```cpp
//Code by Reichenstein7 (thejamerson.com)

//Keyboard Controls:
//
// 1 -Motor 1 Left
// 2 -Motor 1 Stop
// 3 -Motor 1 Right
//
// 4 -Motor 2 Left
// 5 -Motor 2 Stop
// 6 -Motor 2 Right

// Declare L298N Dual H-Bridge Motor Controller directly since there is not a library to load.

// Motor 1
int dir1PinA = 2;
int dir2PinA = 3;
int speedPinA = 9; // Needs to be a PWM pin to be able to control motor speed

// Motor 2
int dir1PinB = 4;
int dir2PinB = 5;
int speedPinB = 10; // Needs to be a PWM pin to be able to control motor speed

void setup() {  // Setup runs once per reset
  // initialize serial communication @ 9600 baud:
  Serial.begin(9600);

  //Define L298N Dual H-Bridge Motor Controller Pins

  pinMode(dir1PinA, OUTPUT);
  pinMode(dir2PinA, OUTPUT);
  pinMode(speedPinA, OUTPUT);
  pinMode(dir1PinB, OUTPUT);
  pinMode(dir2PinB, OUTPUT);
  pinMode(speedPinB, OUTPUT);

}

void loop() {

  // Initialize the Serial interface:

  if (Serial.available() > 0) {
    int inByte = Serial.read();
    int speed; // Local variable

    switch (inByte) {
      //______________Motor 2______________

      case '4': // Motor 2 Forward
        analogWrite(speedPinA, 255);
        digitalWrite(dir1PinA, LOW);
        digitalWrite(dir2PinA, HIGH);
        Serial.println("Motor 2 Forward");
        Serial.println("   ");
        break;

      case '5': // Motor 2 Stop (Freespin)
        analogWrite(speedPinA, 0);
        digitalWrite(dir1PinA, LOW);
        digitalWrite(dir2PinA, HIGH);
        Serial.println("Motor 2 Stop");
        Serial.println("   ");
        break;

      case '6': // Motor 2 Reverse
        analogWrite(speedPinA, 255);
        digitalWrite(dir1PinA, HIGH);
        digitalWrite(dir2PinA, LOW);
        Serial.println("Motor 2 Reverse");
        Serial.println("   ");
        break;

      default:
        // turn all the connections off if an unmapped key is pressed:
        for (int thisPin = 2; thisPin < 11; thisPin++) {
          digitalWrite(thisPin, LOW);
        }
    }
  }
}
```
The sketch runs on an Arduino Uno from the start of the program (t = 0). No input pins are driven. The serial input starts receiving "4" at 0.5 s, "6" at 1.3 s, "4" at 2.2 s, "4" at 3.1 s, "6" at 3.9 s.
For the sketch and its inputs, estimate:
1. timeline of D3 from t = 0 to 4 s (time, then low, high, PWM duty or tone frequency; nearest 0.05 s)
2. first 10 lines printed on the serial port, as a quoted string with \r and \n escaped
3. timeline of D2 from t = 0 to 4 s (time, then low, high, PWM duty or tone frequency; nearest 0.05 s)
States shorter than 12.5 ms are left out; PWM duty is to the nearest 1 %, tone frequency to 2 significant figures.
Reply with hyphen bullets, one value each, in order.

- 0 s low; 0.5 s high; 1.3 s low; 2.2 s high; 3.9 s low
- "Motor 2 Forward\r\n   \r\nMotor 2 Reverse\r\n   \r\nMotor 2 Forward\r\n   \r\nMotor 2 Forward\r\n   \r\nMotor 2 Reverse\r\n   \r\n"
- 0 s low; 1.3 s high; 2.2 s low; 3.9 s high
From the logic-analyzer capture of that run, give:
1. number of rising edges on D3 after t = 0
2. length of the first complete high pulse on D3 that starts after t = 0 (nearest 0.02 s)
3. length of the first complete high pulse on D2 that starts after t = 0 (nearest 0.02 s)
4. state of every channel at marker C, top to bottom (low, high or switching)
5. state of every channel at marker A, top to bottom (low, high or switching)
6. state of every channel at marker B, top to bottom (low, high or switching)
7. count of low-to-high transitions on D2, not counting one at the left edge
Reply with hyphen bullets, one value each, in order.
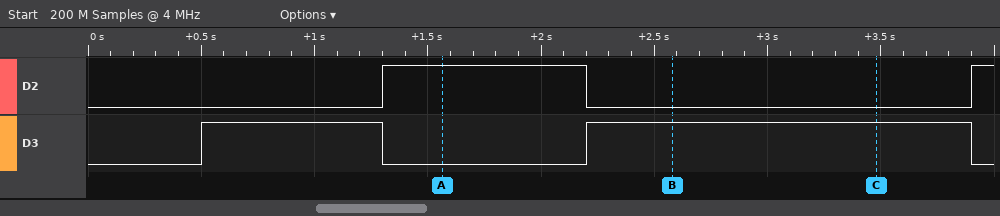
- 2
- 0.80 s
- 0.90 s
- D2 low, D3 high
- D2 high, D3 low
- D2 low, D3 high
- 2
